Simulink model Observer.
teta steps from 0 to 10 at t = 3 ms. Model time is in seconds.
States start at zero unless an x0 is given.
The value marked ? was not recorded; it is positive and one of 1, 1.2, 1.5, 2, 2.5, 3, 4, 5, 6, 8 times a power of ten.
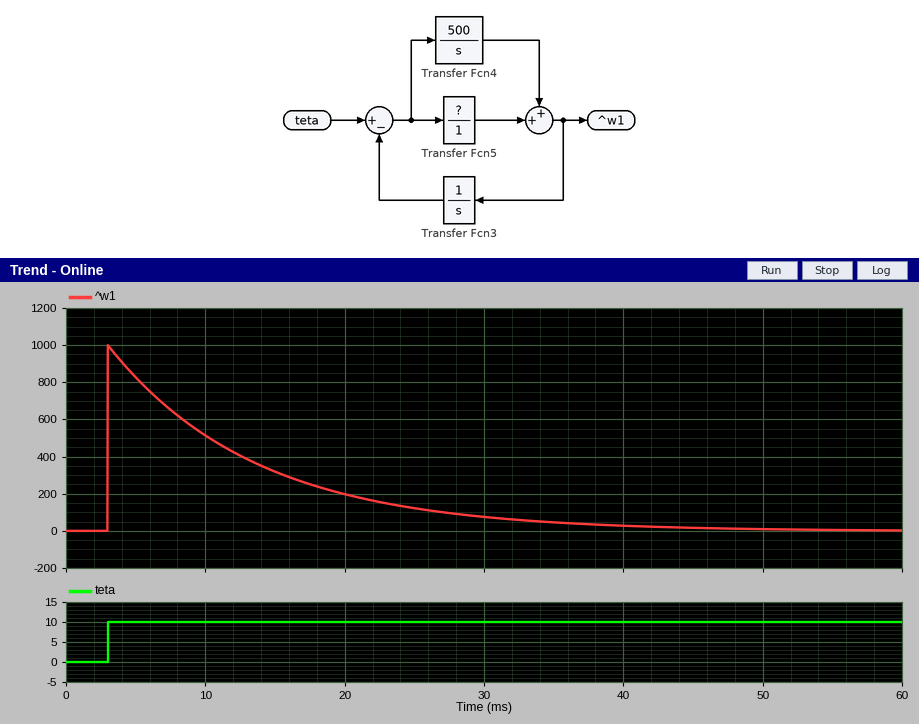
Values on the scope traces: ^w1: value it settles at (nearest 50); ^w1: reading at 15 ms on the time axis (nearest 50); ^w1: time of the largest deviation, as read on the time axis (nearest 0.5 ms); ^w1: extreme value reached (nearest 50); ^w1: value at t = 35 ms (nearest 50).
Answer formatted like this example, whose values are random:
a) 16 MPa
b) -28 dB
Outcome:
a) 0
b) 300
c) 3.0 ms
d) 1000
e) 50
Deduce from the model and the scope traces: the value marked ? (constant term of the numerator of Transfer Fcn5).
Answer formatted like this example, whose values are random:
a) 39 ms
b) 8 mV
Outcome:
a) 100
